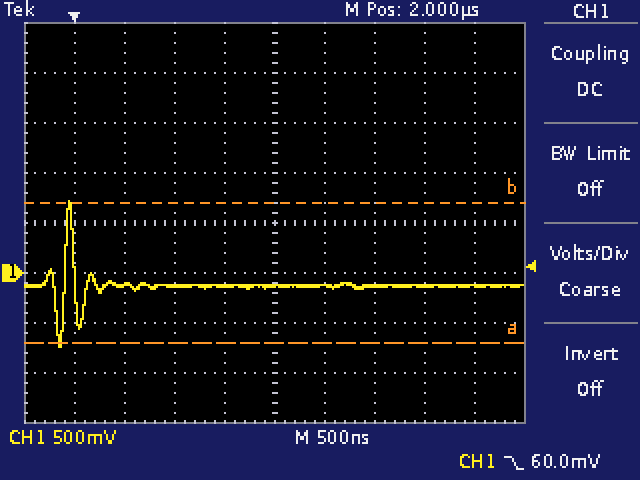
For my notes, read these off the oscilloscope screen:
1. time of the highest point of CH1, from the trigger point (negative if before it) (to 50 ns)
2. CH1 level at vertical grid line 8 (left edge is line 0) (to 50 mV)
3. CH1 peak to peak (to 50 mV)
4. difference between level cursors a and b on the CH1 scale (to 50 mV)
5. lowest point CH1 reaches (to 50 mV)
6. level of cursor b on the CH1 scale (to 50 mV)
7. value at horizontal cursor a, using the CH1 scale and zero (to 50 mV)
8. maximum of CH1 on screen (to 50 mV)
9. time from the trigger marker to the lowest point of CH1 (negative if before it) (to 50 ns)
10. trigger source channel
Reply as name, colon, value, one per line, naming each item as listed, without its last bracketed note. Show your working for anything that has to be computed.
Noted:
time of the highest point of CH1, from the trigger point (negative if before it): -50 ns
CH1 level at vertical grid line 8 (left edge is line 0): -150 mV
CH1 peak to peak: 700 mV − (-750 mV) = 1.45 V
difference between level cursors a and b on the CH1 scale: 1.40 V
lowest point CH1 reaches: -750 mV
level of cursor b on the CH1 scale: 700 mV
value at horizontal cursor a, using the CH1 scale and zero: -700 mV
maximum of CH1 on screen: 700 mV
time from the trigger marker to the lowest point of CH1 (negative if before it): -150 ns
trigger source channel: CH1
